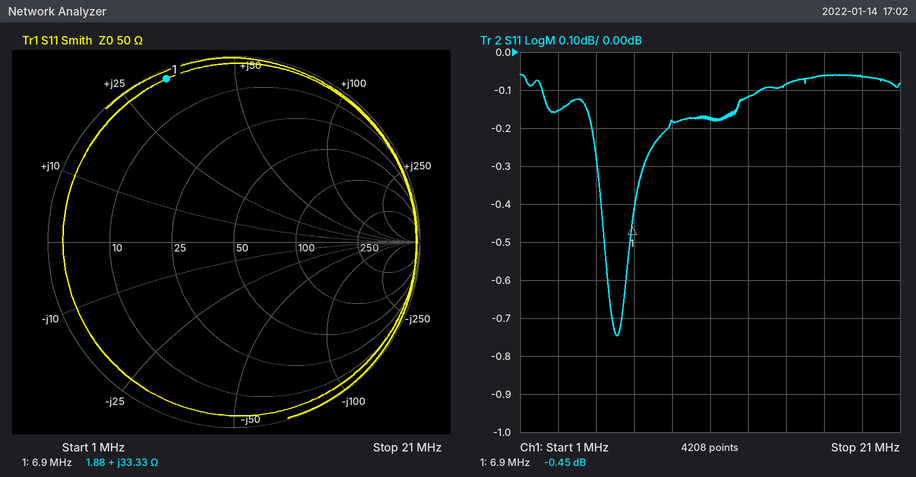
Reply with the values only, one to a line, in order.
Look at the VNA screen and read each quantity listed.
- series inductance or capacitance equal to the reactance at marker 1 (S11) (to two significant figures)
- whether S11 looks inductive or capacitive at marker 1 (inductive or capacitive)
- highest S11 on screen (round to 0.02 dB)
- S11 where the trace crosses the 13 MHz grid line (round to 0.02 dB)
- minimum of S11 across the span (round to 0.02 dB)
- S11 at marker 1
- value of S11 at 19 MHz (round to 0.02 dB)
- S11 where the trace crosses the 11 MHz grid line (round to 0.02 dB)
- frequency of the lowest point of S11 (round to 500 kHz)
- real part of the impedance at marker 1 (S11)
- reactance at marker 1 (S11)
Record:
770 nH
inductive
-0.06 dB
-0.12 dB
-0.74 dB
-0.45 dB
-0.06 dB
-0.18 dB
6.0 MHz
1.88 Ω
+33.33 Ω
